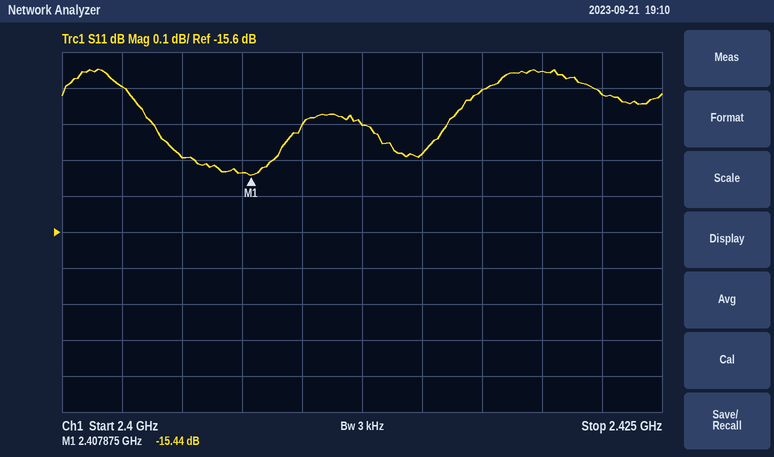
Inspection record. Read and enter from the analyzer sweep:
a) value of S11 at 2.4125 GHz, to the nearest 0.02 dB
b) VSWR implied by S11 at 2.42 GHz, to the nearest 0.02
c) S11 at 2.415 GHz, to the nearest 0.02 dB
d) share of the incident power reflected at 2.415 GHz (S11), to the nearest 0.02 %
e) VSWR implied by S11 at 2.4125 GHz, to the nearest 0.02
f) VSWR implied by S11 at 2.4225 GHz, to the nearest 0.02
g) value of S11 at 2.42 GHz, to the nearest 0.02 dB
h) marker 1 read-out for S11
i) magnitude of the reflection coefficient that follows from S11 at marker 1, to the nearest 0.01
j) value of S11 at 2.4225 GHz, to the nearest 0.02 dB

-15.30 dB
1.42
-15.38 dB
2.90 %
1.42
1.42
-15.16 dB
-15.44 dB
0.17
-15.22 dB
